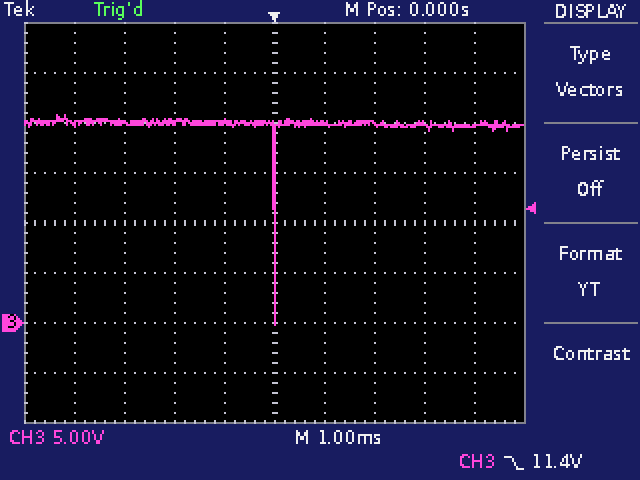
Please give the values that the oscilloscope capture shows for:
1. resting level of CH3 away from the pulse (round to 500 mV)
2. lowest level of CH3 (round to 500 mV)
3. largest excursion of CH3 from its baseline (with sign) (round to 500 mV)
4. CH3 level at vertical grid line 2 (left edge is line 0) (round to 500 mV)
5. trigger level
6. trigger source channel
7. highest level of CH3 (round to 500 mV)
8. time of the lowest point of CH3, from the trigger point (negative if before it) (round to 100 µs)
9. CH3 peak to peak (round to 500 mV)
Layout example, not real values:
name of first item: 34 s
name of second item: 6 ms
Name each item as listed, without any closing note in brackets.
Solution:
resting level of CH3 away from the pulse: 20.0 V
lowest level of CH3: 0.0 V
largest excursion of CH3 from its baseline (with sign): -20.0 V
CH3 level at vertical grid line 2 (left edge is line 0): 20.0 V
trigger level: 11.4 V
trigger source channel: CH3
highest level of CH3: 21.0 V
time of the lowest point of CH3, from the trigger point (negative if before it): 0.0 ms
CH3 peak to peak: 21.0 V
